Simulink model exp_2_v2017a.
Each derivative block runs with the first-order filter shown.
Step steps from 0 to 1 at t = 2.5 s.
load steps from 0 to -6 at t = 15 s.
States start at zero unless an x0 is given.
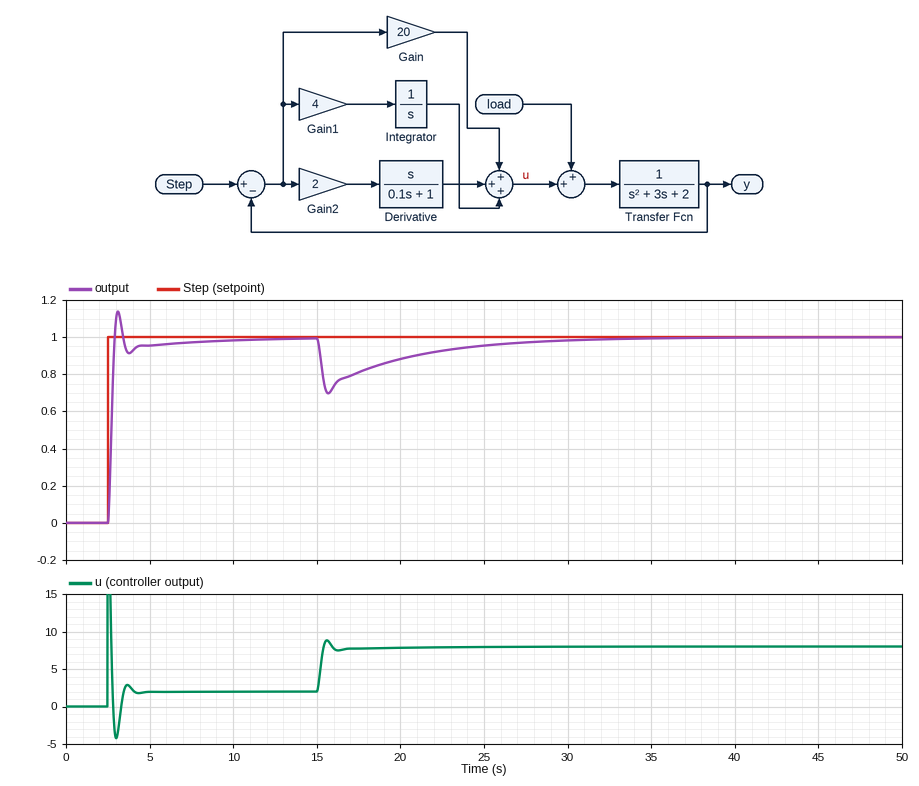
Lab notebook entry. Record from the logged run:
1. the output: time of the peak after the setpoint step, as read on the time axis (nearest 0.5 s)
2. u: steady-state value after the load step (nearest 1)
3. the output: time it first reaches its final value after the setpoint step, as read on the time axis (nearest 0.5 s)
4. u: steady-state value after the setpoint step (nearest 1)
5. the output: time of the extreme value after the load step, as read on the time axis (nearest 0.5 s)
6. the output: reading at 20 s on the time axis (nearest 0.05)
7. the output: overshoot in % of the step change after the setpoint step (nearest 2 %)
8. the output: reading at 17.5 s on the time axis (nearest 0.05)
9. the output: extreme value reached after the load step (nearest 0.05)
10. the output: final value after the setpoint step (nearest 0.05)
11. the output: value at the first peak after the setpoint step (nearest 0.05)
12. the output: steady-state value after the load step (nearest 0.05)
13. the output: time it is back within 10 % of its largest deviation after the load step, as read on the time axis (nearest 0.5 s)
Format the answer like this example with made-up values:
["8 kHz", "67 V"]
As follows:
["3.0 s", "8", "3.0 s", "2", "15.5 s", "0.90", "14 %", "0.80", "0.70", "1.00", "1.15", "1.00", "27.5 s"]
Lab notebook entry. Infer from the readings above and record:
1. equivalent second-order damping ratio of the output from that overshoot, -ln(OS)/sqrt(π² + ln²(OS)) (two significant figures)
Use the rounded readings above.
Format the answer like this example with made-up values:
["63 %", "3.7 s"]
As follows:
["0.53"]
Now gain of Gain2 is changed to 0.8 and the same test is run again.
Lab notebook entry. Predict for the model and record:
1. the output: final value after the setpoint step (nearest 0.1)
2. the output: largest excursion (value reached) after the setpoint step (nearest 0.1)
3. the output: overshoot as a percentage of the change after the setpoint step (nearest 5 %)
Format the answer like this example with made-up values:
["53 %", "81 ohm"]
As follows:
["1.0", "1.2", "20 %"]
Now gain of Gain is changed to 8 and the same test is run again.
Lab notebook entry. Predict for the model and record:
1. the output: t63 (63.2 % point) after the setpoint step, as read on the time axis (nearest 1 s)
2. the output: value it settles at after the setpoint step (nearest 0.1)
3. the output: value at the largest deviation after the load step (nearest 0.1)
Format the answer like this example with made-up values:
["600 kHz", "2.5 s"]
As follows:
["3 s", "1.0", "0.5"]
